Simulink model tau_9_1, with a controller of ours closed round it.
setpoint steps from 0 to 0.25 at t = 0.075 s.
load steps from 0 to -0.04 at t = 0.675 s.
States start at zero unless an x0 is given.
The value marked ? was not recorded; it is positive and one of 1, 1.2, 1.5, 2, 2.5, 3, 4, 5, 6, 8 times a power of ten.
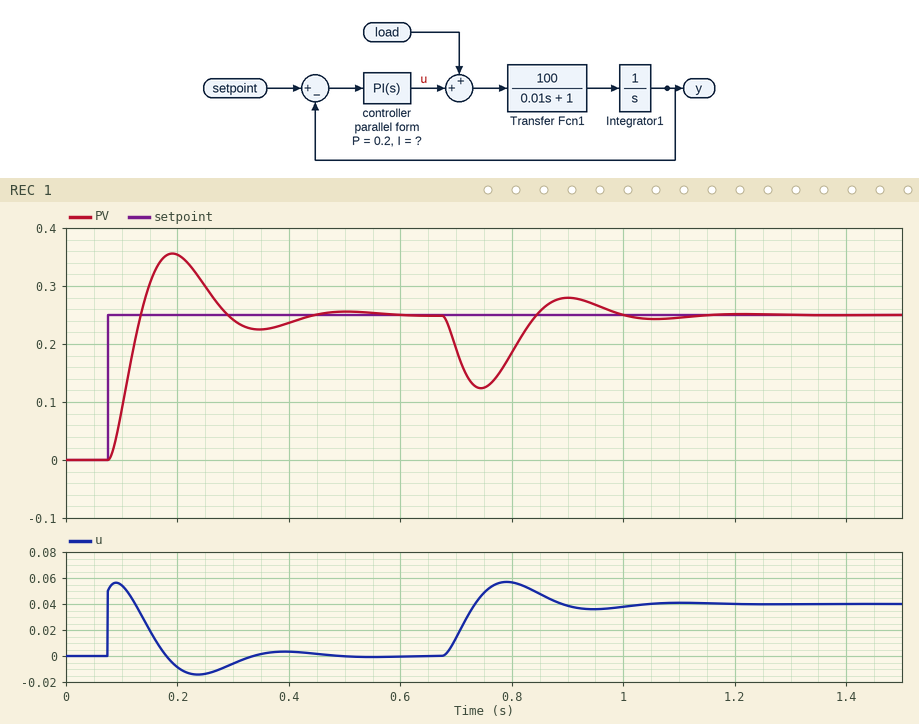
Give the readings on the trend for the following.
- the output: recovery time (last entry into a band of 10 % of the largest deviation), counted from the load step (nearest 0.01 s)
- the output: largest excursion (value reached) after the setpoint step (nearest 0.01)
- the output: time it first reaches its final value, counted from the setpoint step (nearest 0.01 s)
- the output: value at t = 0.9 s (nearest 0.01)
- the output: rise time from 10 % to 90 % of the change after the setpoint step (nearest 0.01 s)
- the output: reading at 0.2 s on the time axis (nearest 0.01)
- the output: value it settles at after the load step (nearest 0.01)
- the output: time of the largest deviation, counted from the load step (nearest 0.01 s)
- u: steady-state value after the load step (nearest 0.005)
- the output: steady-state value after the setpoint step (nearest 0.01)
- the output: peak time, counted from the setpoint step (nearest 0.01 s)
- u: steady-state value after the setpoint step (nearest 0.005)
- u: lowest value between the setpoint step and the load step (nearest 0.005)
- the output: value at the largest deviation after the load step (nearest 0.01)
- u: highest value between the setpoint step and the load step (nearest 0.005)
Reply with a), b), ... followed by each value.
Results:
a) 0.29 s
b) 0.36
c) 0.06 s
d) 0.28
e) 0.04 s
f) 0.35
g) 0.25
h) 0.07 s
i) 0.040
j) 0.25
k) 0.12 s
l) 0.000
m) -0.015
n) 0.12
o) 0.055
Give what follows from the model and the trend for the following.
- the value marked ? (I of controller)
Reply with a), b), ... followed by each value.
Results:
a) 4
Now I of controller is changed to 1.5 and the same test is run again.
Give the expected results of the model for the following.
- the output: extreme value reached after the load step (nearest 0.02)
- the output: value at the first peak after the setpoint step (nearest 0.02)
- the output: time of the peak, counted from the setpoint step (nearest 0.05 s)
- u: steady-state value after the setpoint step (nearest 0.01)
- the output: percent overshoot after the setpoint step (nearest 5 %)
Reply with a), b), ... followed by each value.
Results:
a) 0.10
b) 0.30
c) 0.15 s
d) 0.00
e) 20 %
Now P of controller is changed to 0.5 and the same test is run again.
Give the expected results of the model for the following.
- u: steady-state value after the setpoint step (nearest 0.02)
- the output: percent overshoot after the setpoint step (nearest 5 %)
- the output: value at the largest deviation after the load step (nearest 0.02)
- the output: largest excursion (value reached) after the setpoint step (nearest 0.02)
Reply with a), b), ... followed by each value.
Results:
a) 0.00
b) 20 %
c) 0.18
d) 0.30
